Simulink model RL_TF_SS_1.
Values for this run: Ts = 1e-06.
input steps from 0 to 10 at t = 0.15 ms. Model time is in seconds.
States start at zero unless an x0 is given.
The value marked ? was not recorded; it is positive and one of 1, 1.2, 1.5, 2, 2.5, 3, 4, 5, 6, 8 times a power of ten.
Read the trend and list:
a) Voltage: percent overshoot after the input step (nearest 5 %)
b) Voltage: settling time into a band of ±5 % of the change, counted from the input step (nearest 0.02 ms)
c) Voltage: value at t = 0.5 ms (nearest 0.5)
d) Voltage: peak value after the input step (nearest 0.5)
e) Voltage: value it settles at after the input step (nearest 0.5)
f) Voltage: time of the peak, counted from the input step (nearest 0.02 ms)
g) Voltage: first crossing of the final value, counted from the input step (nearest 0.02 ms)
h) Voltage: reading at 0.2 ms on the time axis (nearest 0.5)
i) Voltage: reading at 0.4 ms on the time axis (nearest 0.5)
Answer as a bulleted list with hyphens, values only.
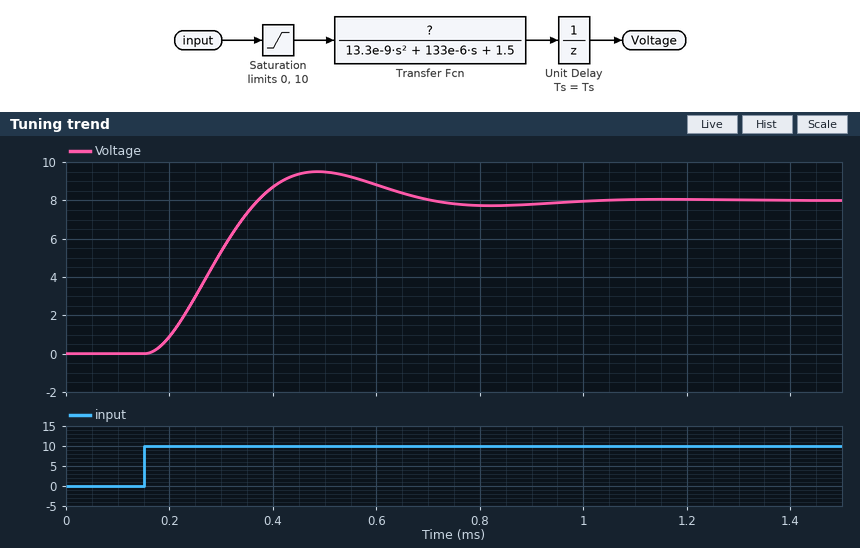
- 20 %
- 0.50 ms
- 9.5
- 9.5
- 8.0
- 0.34 ms
- 0.22 ms
- 1.0
- 8.5
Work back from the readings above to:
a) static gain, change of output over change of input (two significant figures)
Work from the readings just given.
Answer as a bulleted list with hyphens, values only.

- 0.80
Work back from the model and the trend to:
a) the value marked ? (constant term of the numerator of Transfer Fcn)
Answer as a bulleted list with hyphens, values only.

- 1.2
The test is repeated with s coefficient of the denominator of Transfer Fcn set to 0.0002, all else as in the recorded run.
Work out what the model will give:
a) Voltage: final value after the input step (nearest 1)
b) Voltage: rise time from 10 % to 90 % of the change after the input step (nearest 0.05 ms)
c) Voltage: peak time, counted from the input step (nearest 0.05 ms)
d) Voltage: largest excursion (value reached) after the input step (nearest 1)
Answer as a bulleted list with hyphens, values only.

- 8
- 0.20 ms
- 0.40 ms
- 8
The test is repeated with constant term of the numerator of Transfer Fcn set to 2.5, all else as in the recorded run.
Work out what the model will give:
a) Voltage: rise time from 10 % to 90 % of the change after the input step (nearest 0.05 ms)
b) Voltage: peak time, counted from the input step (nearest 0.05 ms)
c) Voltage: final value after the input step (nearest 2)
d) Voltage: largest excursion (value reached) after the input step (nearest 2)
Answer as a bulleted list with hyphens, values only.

- 0.15 ms
- 0.35 ms
- 16
- 20
